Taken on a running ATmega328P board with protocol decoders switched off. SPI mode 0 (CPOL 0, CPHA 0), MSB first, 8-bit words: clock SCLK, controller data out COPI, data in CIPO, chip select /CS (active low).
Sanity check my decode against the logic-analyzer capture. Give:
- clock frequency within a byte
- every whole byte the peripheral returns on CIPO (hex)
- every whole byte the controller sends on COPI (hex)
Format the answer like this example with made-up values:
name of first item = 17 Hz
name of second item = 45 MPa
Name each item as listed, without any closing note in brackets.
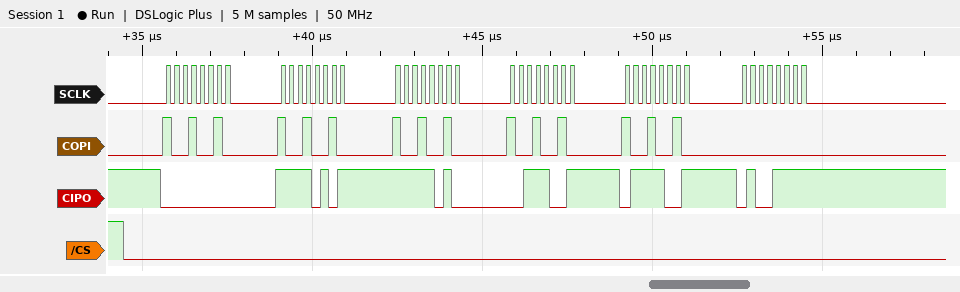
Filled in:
clock frequency within a byte = 4 MHz
every whole byte the peripheral returns on CIPO = 00 F5 FA 39 79 4F
every whole byte the controller sends on COPI = 92 92 92 92 92 00
